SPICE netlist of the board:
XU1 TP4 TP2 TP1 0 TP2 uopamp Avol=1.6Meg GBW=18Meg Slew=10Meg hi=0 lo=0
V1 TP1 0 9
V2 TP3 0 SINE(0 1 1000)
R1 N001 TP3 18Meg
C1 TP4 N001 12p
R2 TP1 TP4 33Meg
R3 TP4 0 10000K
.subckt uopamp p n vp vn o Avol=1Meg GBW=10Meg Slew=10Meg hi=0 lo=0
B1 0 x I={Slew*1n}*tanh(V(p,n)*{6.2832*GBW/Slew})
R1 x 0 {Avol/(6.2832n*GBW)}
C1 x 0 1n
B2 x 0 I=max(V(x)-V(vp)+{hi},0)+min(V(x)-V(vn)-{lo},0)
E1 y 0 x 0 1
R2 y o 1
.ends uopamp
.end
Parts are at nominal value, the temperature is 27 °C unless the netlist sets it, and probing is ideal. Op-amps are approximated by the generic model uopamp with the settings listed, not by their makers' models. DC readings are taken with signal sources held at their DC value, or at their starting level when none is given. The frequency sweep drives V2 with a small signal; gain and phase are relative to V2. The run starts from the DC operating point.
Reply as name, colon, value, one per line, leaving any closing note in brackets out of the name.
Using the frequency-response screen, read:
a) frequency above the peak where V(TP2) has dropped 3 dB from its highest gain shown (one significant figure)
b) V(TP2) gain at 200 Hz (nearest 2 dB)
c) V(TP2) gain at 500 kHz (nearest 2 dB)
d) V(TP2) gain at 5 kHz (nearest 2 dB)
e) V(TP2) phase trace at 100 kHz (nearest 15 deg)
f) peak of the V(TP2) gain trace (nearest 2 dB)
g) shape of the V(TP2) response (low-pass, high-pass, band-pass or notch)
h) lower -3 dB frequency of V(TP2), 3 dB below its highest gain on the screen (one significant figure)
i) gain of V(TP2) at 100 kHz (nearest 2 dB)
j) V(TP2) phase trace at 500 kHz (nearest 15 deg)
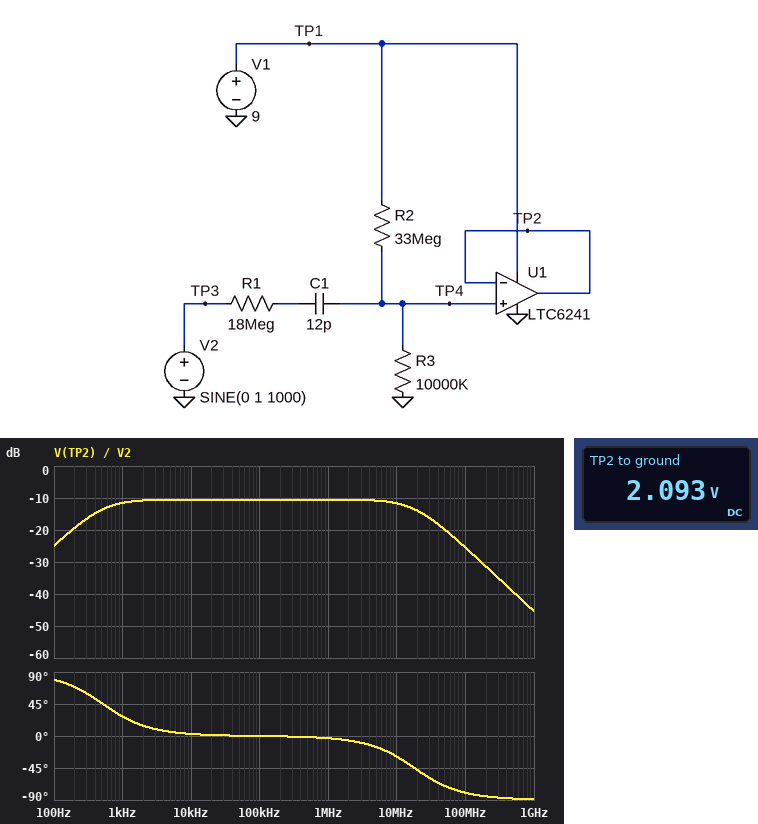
frequency above the peak where V(TP2) has dropped 3 dB from its highest gain shown: 20 MHz
V(TP2) gain at 200 Hz: -20 dB
V(TP2) gain at 500 kHz: -10 dB
V(TP2) gain at 5 kHz: -10 dB
V(TP2) phase trace at 100 kHz: 0 deg
peak of the V(TP2) gain trace: -10 dB
shape of the V(TP2) response: band-pass
lower -3 dB frequency of V(TP2), 3 dB below its highest gain on the screen: 500 Hz
gain of V(TP2) at 100 kHz: -10 dB
V(TP2) phase trace at 500 kHz: 0 deg
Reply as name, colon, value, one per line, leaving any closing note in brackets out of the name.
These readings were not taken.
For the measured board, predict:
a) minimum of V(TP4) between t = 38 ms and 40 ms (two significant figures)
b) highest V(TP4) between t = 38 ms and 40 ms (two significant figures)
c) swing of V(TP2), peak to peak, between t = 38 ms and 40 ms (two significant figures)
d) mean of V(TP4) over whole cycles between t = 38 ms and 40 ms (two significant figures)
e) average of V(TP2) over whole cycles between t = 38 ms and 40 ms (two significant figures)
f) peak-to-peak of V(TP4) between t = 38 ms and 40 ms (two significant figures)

minimum of V(TP4) between t = 38 ms and 40 ms: 1.8 V
highest V(TP4) between t = 38 ms and 40 ms: 2.4 V
swing of V(TP2), peak to peak, between t = 38 ms and 40 ms: 530 mV
mean of V(TP4) over whole cycles between t = 38 ms and 40 ms: 2.1 V
average of V(TP2) over whole cycles between t = 38 ms and 40 ms: 2.1 V
peak-to-peak of V(TP4) between t = 38 ms and 40 ms: 530 mV
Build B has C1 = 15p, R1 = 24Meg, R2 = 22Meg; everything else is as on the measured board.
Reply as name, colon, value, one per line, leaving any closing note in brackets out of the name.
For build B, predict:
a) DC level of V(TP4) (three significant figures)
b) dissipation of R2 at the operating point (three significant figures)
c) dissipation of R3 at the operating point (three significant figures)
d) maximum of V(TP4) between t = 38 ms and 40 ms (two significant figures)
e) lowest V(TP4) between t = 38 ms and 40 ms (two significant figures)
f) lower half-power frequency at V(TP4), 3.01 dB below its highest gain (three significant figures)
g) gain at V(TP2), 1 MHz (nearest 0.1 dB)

DC level of V(TP4): 2.81 V
dissipation of R2 at the operating point: 1.74 µW
dissipation of R3 at the operating point: 791 nW
maximum of V(TP4) between t = 38 ms and 40 ms: 3.0 V
lowest V(TP4) between t = 38 ms and 40 ms: 2.6 V
lower half-power frequency at V(TP4), 3.01 dB below its highest gain: 344 Hz
gain at V(TP2), 1 MHz: -13.1 dB
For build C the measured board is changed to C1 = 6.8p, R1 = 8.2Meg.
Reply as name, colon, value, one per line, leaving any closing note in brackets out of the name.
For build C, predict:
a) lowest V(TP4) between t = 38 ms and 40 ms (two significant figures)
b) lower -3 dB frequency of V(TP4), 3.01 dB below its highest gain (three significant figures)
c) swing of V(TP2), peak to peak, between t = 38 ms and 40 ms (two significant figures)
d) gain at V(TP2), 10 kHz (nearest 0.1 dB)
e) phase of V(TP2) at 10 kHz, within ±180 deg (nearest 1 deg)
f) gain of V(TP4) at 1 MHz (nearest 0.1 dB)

lowest V(TP4) between t = 38 ms and 40 ms: 1.8 V
lower -3 dB frequency of V(TP4), 3.01 dB below its highest gain: 1.47 kHz
swing of V(TP2), peak to peak, between t = 38 ms and 40 ms: 540 mV
gain at V(TP2), 10 kHz: -6.4 dB
phase of V(TP2) at 10 kHz, within ±180 deg: 8 deg
gain of V(TP4) at 1 MHz: -6.3 dB
